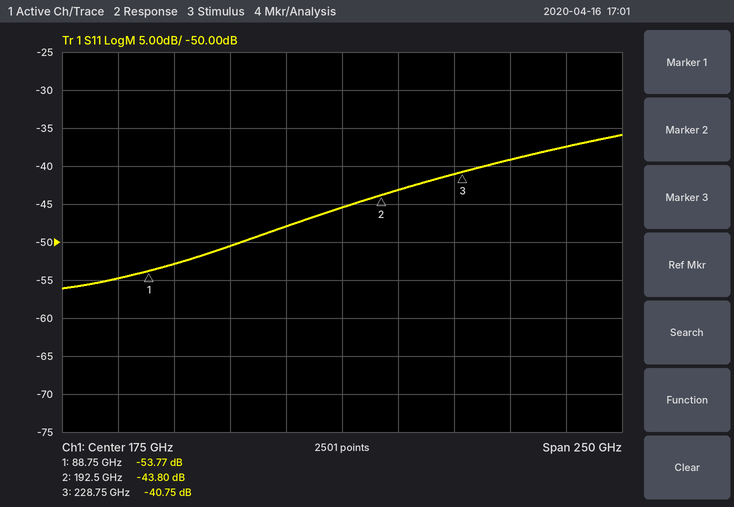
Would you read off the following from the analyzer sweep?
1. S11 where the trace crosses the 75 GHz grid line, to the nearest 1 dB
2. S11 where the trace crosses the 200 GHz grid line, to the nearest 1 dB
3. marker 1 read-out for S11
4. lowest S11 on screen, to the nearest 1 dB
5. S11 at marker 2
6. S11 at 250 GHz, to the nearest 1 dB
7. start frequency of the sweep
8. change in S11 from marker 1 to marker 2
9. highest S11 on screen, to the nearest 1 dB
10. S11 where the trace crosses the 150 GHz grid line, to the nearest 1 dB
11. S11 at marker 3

-55 dB
-43 dB
-53.77 dB
-56 dB
-43.80 dB
-39 dB
50 GHz
9.97 dB
-36 dB
-48 dB
-40.75 dB
